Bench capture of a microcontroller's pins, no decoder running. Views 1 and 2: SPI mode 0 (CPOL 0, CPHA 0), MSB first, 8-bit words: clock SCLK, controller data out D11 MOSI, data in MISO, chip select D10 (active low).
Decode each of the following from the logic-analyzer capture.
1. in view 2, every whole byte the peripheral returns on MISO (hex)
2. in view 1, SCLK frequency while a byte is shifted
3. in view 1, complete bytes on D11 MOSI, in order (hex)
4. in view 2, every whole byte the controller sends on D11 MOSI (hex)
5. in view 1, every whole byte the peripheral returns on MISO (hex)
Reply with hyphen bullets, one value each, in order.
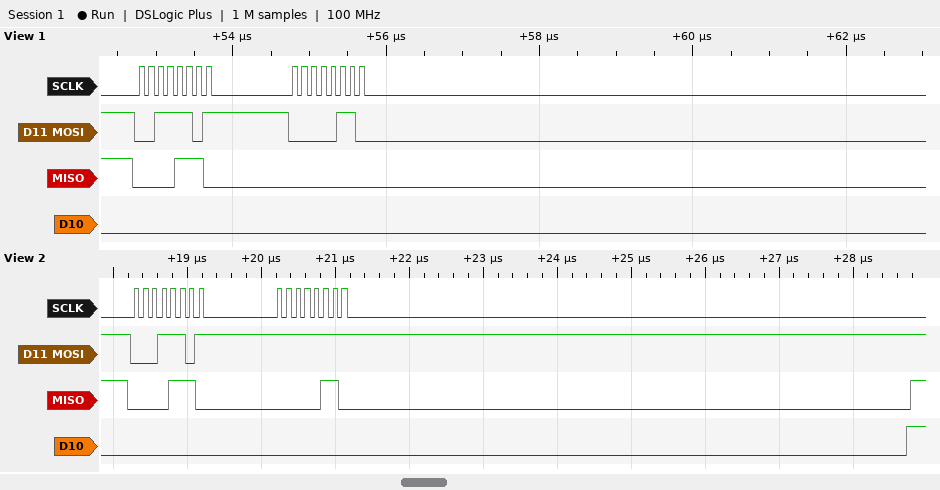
- 0x0E 0x06
- 8 MHz
- 3D 06
- 0x1D 0xFF
- 0E 00
